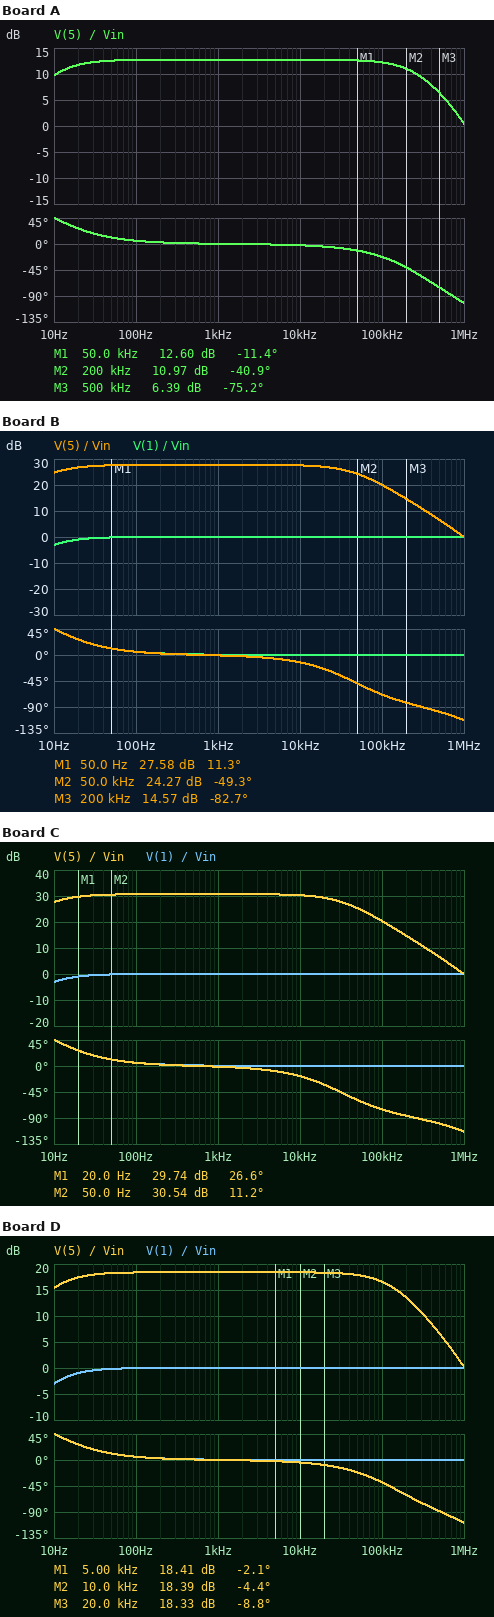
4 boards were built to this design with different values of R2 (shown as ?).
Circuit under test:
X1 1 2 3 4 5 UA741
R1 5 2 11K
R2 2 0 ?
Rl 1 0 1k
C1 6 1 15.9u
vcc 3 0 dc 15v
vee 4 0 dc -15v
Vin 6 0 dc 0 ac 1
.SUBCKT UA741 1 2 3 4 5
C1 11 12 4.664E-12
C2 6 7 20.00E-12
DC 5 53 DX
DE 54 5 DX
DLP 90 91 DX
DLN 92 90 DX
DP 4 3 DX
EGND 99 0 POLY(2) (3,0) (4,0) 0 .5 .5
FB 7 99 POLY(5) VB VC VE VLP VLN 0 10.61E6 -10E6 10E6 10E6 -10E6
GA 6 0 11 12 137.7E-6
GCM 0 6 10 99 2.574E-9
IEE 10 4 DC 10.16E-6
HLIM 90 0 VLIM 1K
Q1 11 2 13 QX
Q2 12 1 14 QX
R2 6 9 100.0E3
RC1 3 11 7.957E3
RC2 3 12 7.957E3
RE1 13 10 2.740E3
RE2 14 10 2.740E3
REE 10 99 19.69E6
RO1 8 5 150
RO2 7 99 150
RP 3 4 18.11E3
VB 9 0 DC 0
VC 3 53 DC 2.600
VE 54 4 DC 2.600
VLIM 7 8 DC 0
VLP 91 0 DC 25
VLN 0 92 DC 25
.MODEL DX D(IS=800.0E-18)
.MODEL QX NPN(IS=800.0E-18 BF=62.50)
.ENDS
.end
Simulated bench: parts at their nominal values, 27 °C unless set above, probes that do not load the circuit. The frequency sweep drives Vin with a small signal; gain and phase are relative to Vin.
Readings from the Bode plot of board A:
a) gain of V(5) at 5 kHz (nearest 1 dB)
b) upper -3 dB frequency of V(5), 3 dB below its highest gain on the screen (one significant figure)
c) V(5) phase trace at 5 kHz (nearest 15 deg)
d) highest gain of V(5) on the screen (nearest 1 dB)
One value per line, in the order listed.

13 dB
300 kHz
0 deg
13 dB
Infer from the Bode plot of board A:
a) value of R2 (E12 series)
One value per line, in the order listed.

3.3 kΩ
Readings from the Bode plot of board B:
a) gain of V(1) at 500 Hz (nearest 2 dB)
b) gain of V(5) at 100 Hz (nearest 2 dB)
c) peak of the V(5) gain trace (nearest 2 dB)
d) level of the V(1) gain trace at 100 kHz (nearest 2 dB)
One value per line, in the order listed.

0 dB
28 dB
28 dB
0 dB
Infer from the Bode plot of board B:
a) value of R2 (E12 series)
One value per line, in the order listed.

470 Ω
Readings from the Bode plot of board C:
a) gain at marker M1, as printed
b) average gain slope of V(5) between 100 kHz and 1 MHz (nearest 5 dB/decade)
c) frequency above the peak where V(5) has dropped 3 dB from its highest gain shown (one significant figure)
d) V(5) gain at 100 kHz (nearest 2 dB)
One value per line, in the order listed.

29.74 dB
-20 dB/decade
30 kHz
20 dB
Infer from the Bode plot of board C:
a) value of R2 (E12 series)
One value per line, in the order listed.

330 Ω
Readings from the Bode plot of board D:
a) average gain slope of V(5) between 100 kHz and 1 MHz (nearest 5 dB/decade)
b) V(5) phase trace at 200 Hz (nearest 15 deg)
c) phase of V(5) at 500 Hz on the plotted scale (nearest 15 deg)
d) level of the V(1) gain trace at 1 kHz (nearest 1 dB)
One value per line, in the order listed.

-15 dB/decade
0 deg
0 deg
0 dB
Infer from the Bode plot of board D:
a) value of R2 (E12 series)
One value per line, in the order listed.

1.5 kΩ
